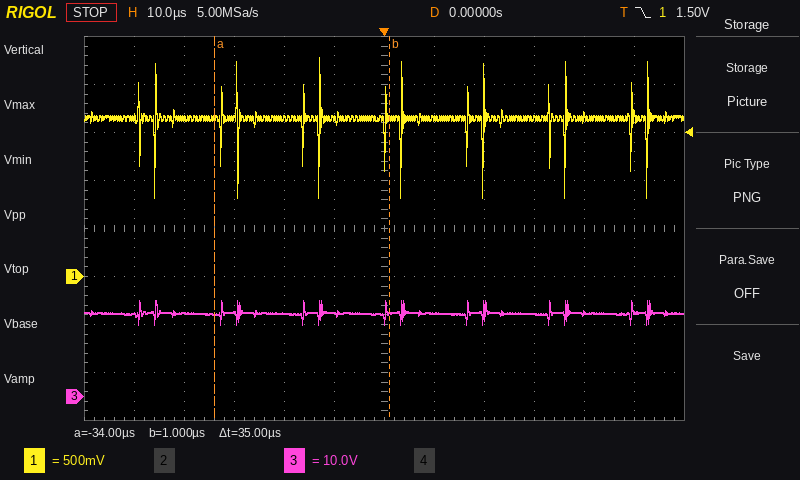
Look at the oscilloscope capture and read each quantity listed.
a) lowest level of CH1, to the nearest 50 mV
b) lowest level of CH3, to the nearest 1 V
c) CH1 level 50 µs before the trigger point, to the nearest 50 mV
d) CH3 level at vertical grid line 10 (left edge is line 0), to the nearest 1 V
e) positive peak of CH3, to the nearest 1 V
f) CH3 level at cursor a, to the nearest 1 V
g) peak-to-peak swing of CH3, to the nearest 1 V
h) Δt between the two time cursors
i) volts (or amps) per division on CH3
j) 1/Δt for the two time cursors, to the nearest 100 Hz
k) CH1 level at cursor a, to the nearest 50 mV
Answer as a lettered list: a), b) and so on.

a) 800 mV
b) 15 V
c) 1.65 V
d) 17 V
e) 20 V
f) 17 V
g) 5 V
h) 35 µs
i) 10 V
j) 28.6 kHz
k) 1.65 V
